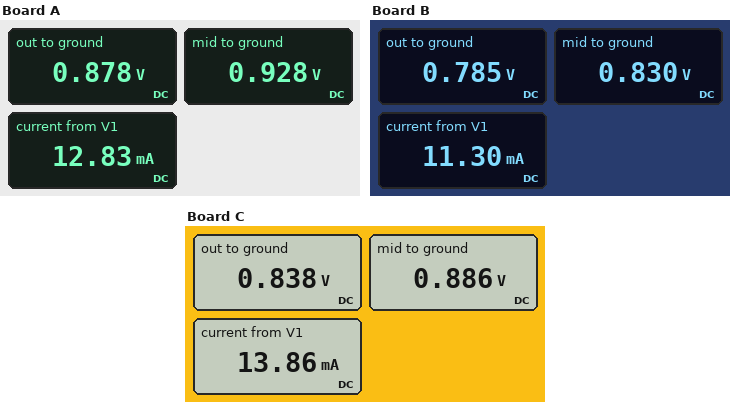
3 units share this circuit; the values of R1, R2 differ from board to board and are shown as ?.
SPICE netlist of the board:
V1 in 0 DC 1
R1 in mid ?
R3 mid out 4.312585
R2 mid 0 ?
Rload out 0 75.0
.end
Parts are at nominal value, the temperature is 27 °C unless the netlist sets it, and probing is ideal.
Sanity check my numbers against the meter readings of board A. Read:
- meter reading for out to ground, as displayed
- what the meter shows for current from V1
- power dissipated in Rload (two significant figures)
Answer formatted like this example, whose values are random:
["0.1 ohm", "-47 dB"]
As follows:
["0.878 V", "12.83 mA", "10 mW"]
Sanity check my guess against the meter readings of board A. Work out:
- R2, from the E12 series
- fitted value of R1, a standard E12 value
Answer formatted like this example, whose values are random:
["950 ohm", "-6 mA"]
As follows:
["820 Ω", "5.6 Ω"]
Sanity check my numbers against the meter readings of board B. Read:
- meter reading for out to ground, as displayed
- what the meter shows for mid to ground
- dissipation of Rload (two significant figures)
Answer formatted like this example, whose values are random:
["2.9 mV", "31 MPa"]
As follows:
["0.785 V", "0.830 V", "8.2 mW"]
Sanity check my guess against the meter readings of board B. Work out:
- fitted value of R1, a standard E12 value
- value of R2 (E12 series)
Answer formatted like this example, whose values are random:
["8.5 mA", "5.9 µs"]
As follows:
["15 Ω", "1 kΩ"]
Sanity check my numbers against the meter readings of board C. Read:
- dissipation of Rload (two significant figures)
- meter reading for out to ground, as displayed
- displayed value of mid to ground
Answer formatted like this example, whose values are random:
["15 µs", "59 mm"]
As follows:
["9.4 mW", "0.838 V", "0.886 V"]
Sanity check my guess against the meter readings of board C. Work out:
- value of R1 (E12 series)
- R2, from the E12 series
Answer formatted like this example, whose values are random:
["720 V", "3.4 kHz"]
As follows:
["8.2 Ω", "330 Ω"]
